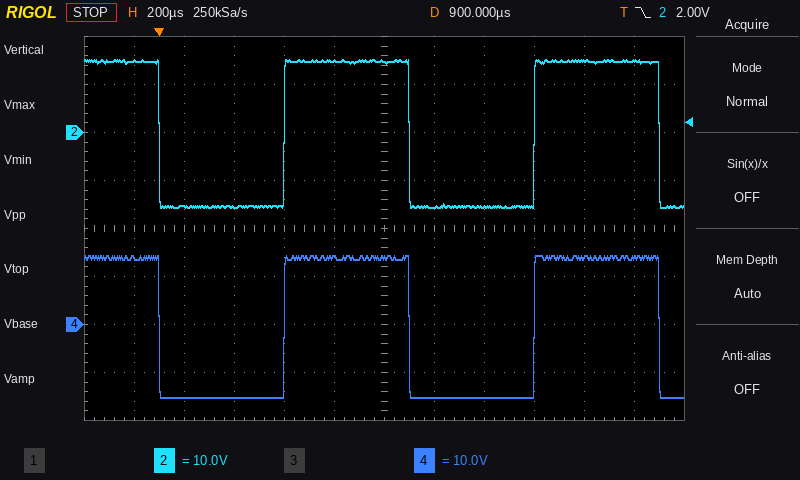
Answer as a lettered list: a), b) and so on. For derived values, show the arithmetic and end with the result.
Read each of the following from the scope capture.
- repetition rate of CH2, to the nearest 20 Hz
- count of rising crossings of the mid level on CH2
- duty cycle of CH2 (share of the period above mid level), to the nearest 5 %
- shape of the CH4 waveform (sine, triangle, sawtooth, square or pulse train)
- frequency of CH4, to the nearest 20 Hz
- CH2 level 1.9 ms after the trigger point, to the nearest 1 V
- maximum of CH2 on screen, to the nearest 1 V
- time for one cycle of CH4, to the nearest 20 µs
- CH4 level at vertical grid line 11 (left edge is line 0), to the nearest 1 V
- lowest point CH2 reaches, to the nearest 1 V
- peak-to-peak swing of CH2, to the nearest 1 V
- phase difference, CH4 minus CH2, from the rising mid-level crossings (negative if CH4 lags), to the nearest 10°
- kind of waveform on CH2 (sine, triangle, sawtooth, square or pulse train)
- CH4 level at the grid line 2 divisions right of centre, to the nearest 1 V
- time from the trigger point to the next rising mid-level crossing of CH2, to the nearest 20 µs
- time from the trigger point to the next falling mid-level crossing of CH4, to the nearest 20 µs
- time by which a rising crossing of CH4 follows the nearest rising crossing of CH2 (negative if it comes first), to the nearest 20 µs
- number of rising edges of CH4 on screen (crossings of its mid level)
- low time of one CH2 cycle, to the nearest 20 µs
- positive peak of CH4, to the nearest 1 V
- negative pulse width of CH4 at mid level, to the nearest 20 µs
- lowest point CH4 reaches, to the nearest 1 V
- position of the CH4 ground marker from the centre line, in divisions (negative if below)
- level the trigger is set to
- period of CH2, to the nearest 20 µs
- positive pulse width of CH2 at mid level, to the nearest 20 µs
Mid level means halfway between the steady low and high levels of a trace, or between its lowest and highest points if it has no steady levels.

a) 1 / 1.00 ms ≈ 1.00 kHz
b) 2
c) 500 µs / 1.00 ms ≈ 50 %
d) square
e) 1 / 1.00 ms ≈ 1.00 kHz
f) 15 V
g) 15 V
h) 1.00 ms
i) 14 V
j) -16 V
k) 15 V − (-16 V) = 31 V
l) −360° × (0 µs) / 1.00 ms ≈ 0°
m) square
n) -15 V
o) 500 µs
p) 1.00 ms
q) 0 µs
r) 2
s) 500 µs
t) 14 V
u) 500 µs
v) -15 V
w) -2.0 div
x) 2.00 V
y) 1.00 ms
z) 500 µs
